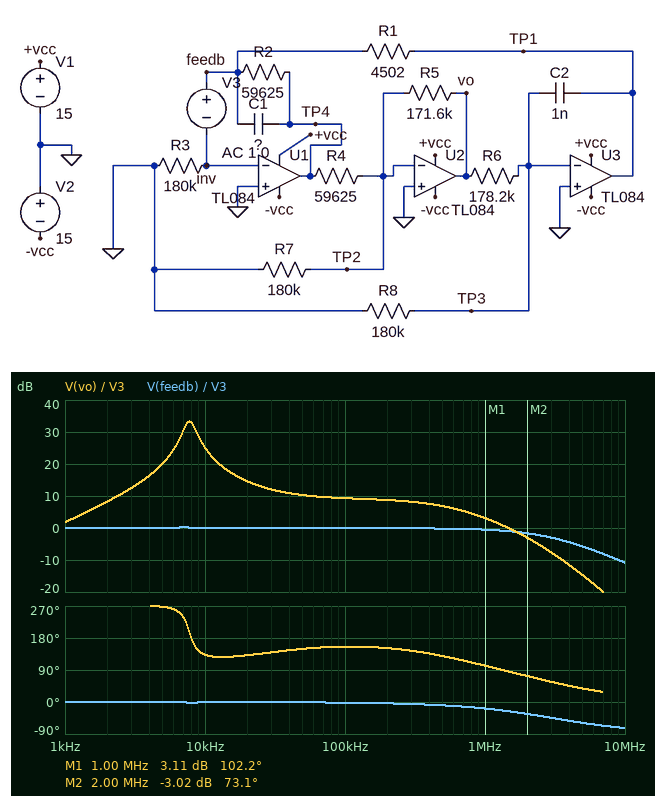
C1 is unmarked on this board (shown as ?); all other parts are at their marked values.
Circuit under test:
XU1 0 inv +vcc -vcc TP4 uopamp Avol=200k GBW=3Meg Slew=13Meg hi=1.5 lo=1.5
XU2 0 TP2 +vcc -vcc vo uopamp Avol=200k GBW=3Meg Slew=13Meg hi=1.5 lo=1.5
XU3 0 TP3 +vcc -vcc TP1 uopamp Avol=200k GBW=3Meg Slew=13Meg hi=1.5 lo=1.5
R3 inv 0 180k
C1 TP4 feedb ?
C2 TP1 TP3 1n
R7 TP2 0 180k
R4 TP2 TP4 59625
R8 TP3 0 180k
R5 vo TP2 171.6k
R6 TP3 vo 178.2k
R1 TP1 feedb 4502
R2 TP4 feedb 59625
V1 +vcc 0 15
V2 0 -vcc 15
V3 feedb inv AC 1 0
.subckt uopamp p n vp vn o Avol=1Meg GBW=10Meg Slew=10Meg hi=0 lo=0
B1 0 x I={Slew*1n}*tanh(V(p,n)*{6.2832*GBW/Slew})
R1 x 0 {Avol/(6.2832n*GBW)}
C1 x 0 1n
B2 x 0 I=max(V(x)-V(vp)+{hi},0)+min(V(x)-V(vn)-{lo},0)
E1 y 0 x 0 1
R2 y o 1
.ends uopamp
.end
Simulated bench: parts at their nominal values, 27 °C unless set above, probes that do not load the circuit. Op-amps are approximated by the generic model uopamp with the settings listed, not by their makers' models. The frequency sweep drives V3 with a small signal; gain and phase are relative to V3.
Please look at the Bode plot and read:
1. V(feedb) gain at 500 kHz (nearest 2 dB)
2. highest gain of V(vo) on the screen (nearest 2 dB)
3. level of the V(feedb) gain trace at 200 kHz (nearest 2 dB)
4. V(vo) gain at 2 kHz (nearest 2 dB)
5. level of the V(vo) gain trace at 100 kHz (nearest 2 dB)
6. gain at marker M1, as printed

0 dB
34 dB
0 dB
8 dB
10 dB
3.11 dB
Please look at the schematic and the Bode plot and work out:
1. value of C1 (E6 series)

1.5 nF
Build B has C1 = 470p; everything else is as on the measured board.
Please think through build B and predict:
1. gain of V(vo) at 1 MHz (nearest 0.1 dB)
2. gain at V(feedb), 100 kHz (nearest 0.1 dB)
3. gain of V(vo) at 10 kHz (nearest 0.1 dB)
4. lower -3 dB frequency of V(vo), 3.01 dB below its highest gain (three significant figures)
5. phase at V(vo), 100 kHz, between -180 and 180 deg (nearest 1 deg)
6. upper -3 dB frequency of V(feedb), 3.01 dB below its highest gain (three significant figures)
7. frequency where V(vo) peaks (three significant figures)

3.0 dB
-0.2 dB
27.0 dB
11.4 kHz
133 deg
2.71 MHz
13.7 kHz
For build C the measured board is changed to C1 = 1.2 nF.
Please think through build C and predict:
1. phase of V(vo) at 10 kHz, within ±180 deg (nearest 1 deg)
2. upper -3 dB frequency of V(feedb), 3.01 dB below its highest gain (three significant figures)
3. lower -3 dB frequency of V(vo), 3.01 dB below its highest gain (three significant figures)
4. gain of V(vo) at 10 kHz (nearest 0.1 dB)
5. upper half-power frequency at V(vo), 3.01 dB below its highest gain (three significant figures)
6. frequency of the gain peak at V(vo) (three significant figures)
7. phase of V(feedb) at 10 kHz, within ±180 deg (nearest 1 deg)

145 deg
2.81 MHz
7.71 kHz
29.3 dB
9.75 kHz
8.66 kHz
-2 deg
